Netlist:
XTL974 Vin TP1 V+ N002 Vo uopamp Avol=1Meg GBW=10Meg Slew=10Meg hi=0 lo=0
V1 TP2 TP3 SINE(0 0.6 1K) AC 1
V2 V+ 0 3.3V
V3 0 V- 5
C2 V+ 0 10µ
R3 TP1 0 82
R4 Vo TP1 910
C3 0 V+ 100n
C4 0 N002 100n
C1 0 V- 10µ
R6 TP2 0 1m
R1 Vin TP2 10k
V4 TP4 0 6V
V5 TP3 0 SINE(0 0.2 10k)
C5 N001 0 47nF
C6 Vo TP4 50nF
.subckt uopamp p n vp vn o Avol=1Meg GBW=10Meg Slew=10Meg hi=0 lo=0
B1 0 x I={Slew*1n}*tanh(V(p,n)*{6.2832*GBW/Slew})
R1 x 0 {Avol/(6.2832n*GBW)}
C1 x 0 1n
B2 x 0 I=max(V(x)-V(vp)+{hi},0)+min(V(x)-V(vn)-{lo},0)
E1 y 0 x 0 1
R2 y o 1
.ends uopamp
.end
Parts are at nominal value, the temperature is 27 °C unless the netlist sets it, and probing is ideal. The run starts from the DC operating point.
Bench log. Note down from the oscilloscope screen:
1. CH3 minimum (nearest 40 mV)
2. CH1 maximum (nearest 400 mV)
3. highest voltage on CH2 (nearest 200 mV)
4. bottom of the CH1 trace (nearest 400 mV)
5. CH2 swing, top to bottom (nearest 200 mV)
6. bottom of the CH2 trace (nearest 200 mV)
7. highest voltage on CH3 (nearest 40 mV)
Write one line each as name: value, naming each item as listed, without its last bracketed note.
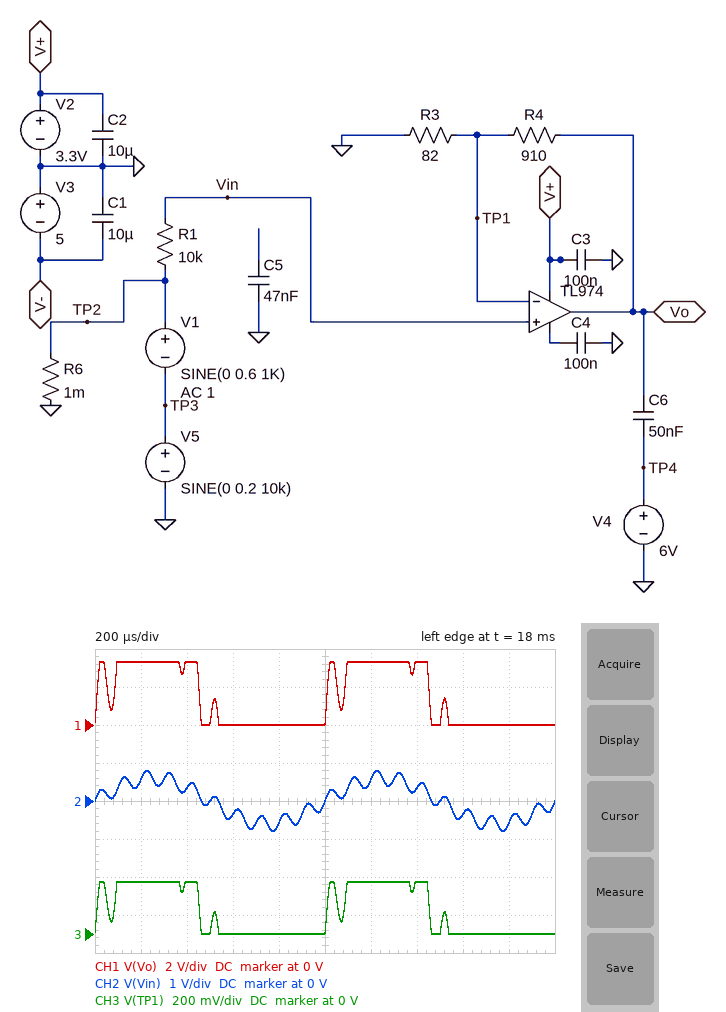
CH3 minimum: 0 V
CH1 maximum: 3.2 V
highest voltage on CH2: 800 mV
bottom of the CH1 trace: 0 V
CH2 swing, top to bottom: 1.6 V
bottom of the CH2 trace: -800 mV
highest voltage on CH3: 280 mV
